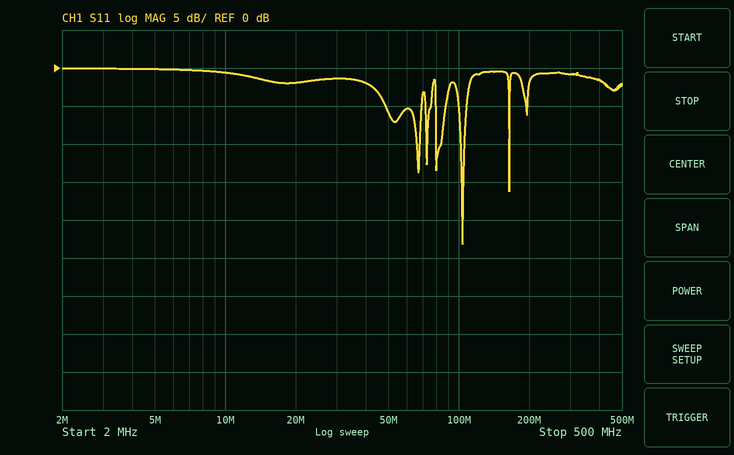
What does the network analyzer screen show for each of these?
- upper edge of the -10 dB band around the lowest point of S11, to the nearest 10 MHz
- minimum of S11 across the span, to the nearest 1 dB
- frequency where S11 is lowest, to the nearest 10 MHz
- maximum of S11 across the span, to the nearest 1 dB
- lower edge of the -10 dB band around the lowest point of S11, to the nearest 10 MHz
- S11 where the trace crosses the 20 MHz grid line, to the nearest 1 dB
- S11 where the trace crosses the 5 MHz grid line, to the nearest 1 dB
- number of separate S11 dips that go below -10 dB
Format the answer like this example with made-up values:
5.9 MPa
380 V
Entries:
110 MHz
-23 dB
100 MHz
0 dB
100 MHz
-2 dB
0 dB
5
